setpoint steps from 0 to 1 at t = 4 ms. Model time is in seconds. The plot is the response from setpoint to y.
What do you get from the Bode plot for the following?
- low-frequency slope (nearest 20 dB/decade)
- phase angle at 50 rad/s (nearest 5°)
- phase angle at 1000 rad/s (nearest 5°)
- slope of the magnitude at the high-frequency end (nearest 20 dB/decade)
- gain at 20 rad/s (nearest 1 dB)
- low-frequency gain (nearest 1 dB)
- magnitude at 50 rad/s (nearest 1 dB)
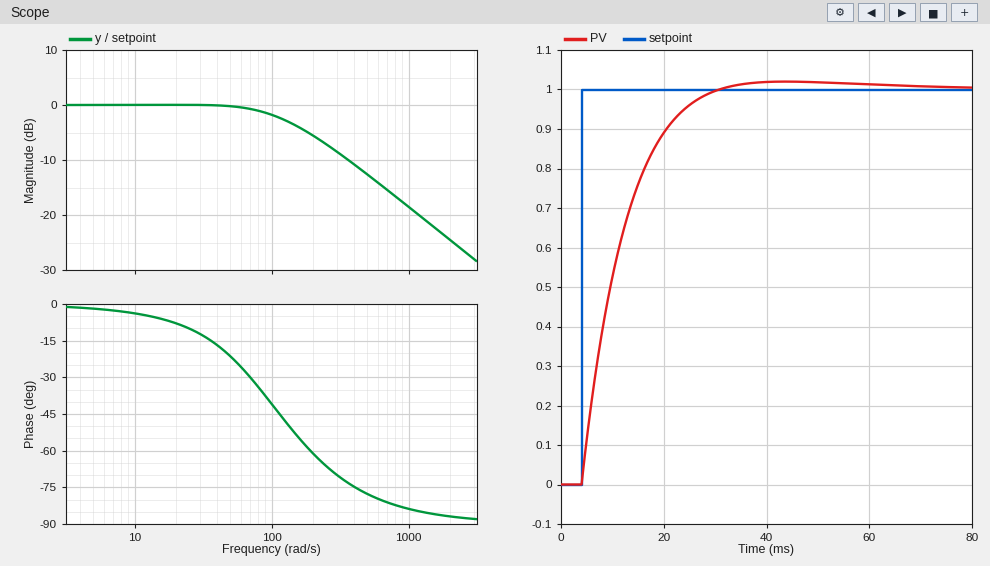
0 dB/decade
-20°
-85°
-20 dB/decade
0 dB
0 dB
0 dB
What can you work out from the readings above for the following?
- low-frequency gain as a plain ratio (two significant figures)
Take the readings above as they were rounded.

1.0
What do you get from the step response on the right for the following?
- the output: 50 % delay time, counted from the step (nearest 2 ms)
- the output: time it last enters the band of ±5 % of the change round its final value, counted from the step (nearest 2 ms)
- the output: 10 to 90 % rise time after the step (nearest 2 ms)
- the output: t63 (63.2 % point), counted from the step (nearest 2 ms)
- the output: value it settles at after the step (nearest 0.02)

6 ms
20 ms
16 ms
8 ms
1.00
